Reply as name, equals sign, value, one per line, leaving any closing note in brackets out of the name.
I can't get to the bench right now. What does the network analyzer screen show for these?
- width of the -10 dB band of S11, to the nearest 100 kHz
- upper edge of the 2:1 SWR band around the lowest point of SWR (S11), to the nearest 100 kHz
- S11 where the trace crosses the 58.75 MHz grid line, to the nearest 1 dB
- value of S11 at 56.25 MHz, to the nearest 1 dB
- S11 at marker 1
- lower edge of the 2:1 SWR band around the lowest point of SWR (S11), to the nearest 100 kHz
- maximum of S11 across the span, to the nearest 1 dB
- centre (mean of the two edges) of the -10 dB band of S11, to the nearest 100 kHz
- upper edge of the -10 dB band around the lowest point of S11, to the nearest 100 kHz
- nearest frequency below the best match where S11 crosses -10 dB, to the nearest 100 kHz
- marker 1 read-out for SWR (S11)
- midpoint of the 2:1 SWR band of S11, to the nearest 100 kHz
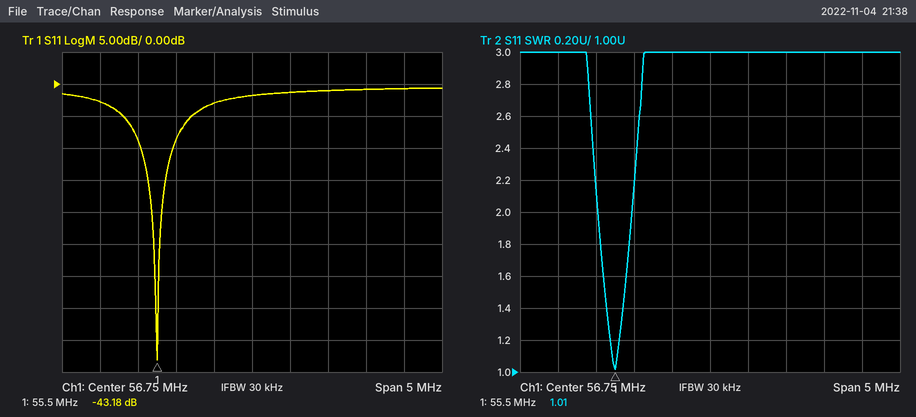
width of the -10 dB band of S11, to the nearest 100 kHz = 400 kHz
upper edge of the 2:1 SWR band around the lowest point of SWR (S11), to the nearest 100 kHz = 55.7 MHz
S11 where the trace crosses the 58.75 MHz grid line, to the nearest 1 dB = -1 dB
value of S11 at 56.25 MHz, to the nearest 1 dB = -3 dB
S11 at marker 1 = -43.18 dB
lower edge of the 2:1 SWR band around the lowest point of SWR (S11), to the nearest 100 kHz = 55.3 MHz
maximum of S11 across the span, to the nearest 1 dB = -1 dB
centre (mean of the two edges) of the -10 dB band of S11, to the nearest 100 kHz = 55.5 MHz
upper edge of the -10 dB band around the lowest point of S11, to the nearest 100 kHz = 55.7 MHz
nearest frequency below the best match where S11 crosses -10 dB, to the nearest 100 kHz = 55.3 MHz
marker 1 read-out for SWR = 1.01
midpoint of the 2:1 SWR band of S11, to the nearest 100 kHz = 55.5 MHz
